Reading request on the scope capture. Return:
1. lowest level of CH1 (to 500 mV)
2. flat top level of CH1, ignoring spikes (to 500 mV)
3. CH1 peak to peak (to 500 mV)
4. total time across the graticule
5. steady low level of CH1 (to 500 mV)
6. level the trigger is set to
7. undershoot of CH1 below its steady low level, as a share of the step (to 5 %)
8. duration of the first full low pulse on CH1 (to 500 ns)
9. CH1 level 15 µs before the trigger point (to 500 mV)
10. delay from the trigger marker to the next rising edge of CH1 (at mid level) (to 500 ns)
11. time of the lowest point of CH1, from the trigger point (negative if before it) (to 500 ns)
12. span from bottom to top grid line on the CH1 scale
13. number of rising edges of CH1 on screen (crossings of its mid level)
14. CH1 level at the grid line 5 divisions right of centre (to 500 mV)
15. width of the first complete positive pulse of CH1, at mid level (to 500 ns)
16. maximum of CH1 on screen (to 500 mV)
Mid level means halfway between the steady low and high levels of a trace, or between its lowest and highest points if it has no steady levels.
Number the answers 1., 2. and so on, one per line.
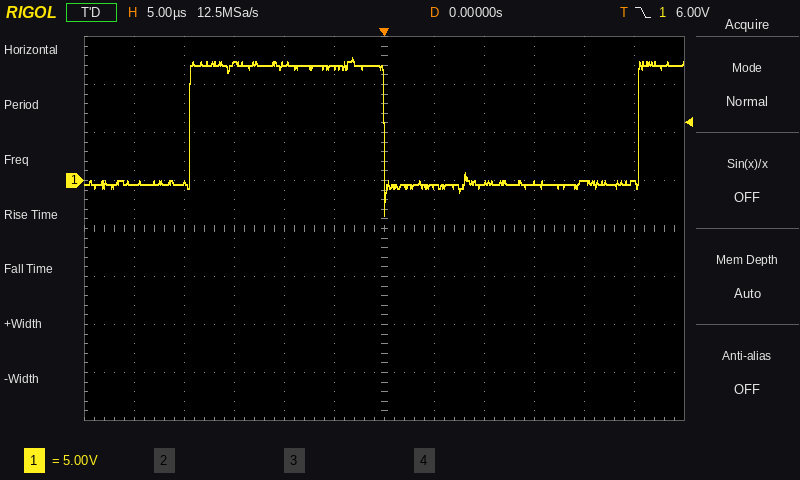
1. -3.5 V
2. 12.0 V
3. 16.5 V
4. 60 µs
5. -500 mV
6. 6.00 V
7. 25 %
8. 25.5 µs
9. 12.0 V
10. 25.5 µs
11. 0.0 µs
12. 40 V
13. 2
14. -500 mV
15. 19.5 µs
16. 13.0 V
